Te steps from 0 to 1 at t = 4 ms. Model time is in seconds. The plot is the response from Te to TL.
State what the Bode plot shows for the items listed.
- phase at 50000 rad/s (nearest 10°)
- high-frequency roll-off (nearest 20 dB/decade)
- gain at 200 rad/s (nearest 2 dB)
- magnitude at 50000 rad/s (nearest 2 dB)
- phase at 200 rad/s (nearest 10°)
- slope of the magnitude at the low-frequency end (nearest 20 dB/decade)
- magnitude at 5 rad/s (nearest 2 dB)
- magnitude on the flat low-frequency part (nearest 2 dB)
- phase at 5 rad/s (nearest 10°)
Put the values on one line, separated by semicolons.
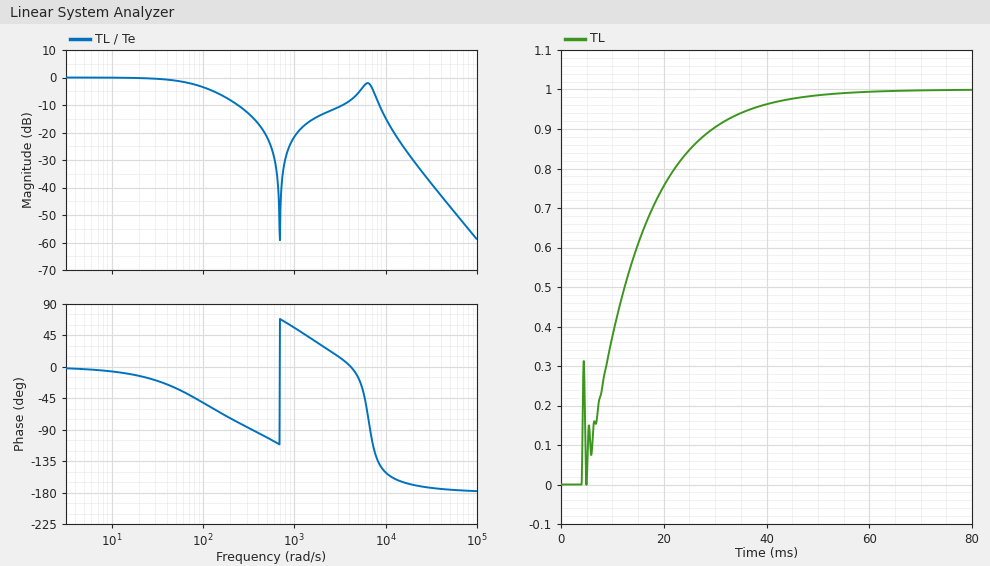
-180°; -40 dB/decade; -8 dB; -46 dB; -70°; 0 dB/decade; 0 dB; 0 dB; 0°
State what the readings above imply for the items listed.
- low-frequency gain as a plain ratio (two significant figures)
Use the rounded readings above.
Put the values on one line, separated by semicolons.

1.0
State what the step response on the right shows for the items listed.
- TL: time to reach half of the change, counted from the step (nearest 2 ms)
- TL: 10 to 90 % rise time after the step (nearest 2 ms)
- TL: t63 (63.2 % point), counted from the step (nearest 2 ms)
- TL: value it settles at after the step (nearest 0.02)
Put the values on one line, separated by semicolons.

8 ms; 26 ms; 12 ms; 1.00
